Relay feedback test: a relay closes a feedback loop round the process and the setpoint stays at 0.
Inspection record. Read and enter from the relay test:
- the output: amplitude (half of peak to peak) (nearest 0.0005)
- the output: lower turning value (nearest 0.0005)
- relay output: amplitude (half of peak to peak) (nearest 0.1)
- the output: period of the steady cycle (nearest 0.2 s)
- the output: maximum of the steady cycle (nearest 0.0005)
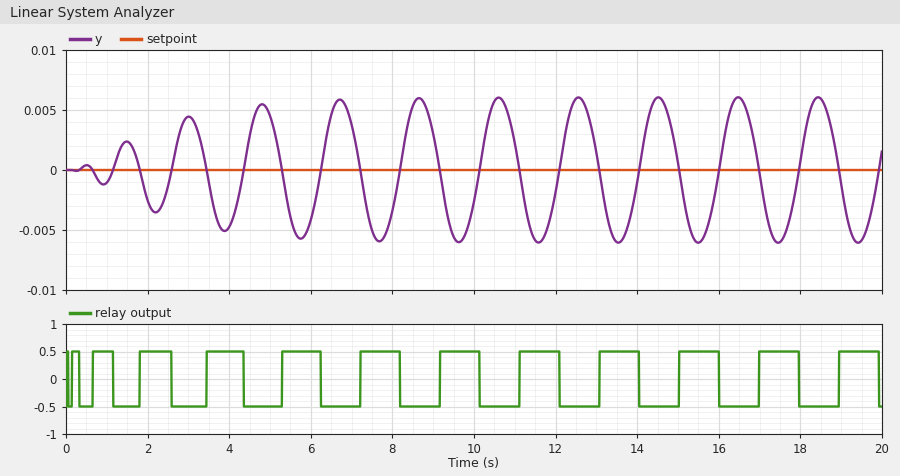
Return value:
0.0060
-0.0060
0.5
2.0 s
0.0060
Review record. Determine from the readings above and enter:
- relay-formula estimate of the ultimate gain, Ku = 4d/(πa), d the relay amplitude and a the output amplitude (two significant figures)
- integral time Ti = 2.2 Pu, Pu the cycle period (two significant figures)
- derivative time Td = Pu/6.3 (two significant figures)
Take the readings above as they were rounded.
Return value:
110
4.4 s
0.32 s
